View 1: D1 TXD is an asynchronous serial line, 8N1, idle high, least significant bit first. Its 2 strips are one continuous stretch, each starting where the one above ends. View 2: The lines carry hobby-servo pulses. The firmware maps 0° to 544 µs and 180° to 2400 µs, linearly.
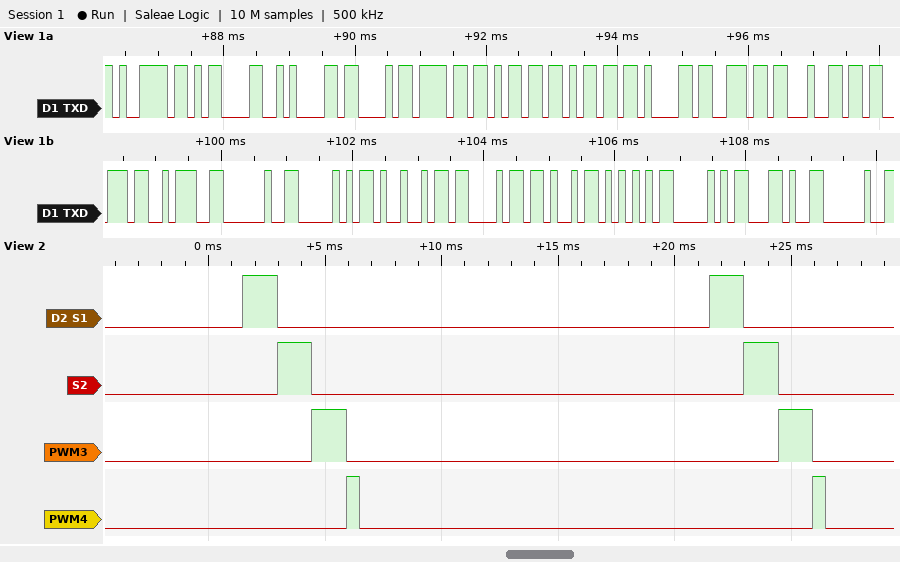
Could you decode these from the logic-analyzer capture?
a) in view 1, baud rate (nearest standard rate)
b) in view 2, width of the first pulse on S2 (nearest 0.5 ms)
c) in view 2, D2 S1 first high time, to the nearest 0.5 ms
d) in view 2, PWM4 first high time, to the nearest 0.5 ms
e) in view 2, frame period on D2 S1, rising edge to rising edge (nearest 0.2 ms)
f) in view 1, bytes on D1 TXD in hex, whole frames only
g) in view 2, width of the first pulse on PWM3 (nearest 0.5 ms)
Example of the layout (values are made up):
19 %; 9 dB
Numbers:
9600 baud; 1.5 ms; 1.5 ms; 0.5 ms; 20.0 ms; 0x79 0x0D 0x0A 0x43 0x6F 0x6D 0x6D 0x61 0x6E 0x64 0x73 0x3A 0x20 0x50 0x49 0x43 0x4B 0x55 0x50 0x2C 0x20; 1.5 ms
